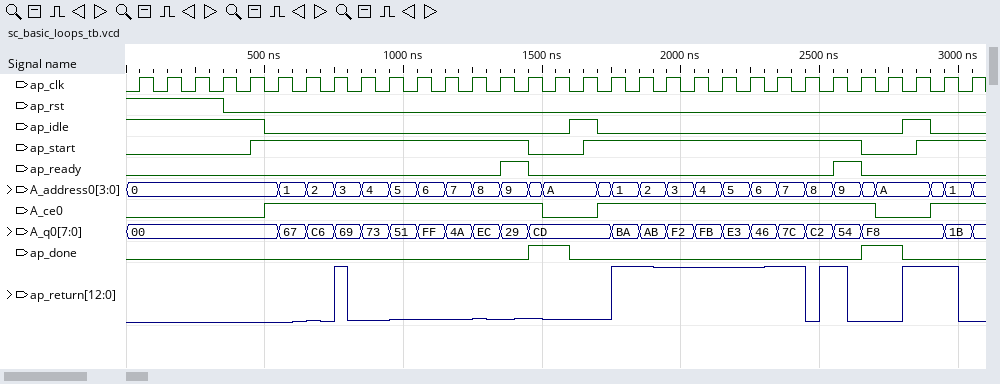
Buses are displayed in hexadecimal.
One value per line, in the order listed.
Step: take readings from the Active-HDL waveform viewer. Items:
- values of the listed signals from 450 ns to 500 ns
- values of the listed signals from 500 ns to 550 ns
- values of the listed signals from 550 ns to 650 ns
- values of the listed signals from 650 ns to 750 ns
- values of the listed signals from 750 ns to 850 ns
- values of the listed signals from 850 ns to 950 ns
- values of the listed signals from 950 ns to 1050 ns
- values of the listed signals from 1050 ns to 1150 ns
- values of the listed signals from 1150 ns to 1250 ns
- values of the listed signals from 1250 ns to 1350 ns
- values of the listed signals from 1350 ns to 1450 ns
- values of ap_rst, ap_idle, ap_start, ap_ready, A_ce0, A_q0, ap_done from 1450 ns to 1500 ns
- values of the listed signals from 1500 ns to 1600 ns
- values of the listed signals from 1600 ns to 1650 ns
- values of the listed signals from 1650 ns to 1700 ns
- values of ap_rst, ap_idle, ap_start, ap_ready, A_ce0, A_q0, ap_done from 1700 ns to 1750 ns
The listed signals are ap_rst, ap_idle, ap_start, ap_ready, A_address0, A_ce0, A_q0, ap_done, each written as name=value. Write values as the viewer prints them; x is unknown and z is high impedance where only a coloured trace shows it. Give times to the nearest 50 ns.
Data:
ap_rst=0, ap_idle=1, ap_start=1, ap_ready=0, A_address0=0, A_ce0=0, A_q0=00, ap_done=0
ap_rst=0, ap_idle=0, ap_start=1, ap_ready=0, A_address0=0, A_ce0=1, A_q0=00, ap_done=0
ap_rst=0, ap_idle=0, ap_start=1, ap_ready=0, A_address0=1, A_ce0=1, A_q0=67, ap_done=0
ap_rst=0, ap_idle=0, ap_start=1, ap_ready=0, A_address0=2, A_ce0=1, A_q0=C6, ap_done=0
ap_rst=0, ap_idle=0, ap_start=1, ap_ready=0, A_address0=3, A_ce0=1, A_q0=69, ap_done=0
ap_rst=0, ap_idle=0, ap_start=1, ap_ready=0, A_address0=4, A_ce0=1, A_q0=73, ap_done=0
ap_rst=0, ap_idle=0, ap_start=1, ap_ready=0, A_address0=5, A_ce0=1, A_q0=51, ap_done=0
ap_rst=0, ap_idle=0, ap_start=1, ap_ready=0, A_address0=6, A_ce0=1, A_q0=FF, ap_done=0
ap_rst=0, ap_idle=0, ap_start=1, ap_ready=0, A_address0=7, A_ce0=1, A_q0=4A, ap_done=0
ap_rst=0, ap_idle=0, ap_start=1, ap_ready=0, A_address0=8, A_ce0=1, A_q0=EC, ap_done=0
ap_rst=0, ap_idle=0, ap_start=1, ap_ready=1, A_address0=9, A_ce0=1, A_q0=29, ap_done=0
ap_rst=0, ap_idle=0, ap_start=0, ap_ready=0, A_ce0=1, A_q0=CD, ap_done=1
ap_rst=0, ap_idle=0, ap_start=0, ap_ready=0, A_address0=A, A_ce0=0, A_q0=CD, ap_done=1
ap_rst=0, ap_idle=1, ap_start=0, ap_ready=0, A_address0=A, A_ce0=0, A_q0=CD, ap_done=0
ap_rst=0, ap_idle=1, ap_start=1, ap_ready=0, A_address0=A, A_ce0=0, A_q0=CD, ap_done=0
ap_rst=0, ap_idle=0, ap_start=1, ap_ready=0, A_ce0=1, A_q0=CD, ap_done=0
